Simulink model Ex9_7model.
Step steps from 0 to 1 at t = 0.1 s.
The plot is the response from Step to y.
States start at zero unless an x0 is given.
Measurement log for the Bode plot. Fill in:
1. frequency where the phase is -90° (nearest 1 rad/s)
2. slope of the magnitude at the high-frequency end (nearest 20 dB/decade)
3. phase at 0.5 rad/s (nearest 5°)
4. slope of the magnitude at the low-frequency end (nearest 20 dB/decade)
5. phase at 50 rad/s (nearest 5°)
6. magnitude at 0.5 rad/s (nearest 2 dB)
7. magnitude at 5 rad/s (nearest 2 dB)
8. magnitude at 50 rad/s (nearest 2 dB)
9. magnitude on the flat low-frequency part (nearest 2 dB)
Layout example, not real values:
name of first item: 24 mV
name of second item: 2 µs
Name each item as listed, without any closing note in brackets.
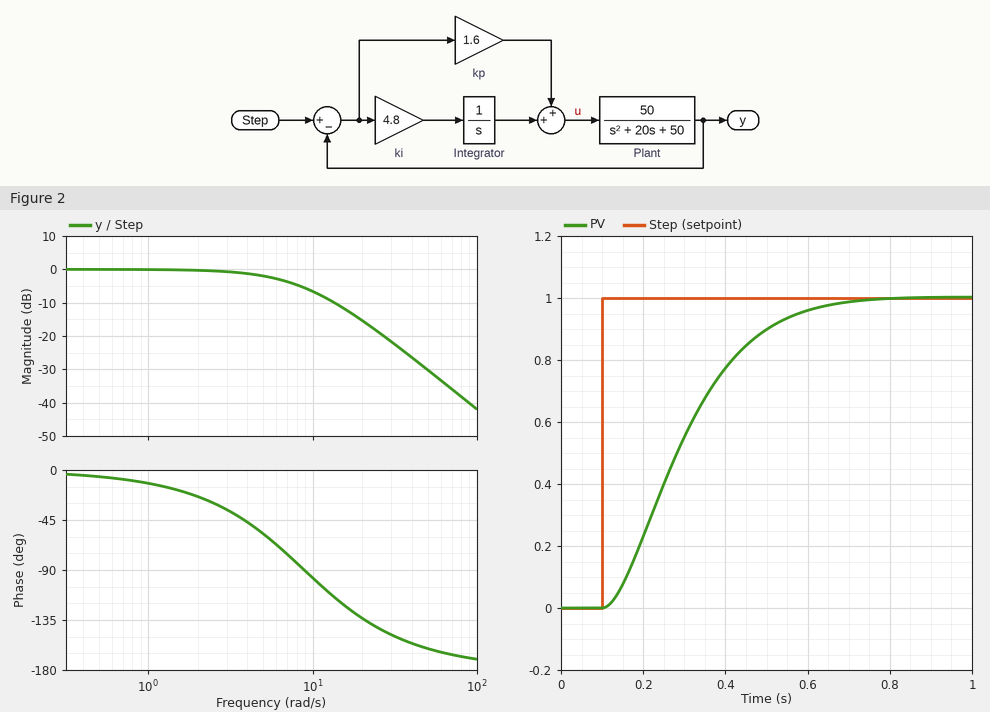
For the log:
frequency where the phase is -90°: 9 rad/s
slope of the magnitude at the high-frequency end: -40 dB/decade
phase at 0.5 rad/s: -5°
slope of the magnitude at the low-frequency end: 0 dB/decade
phase at 50 rad/s: -160°
magnitude at 0.5 rad/s: 0 dB
magnitude at 5 rad/s: -2 dB
magnitude at 50 rad/s: -30 dB
magnitude on the flat low-frequency part: 0 dB
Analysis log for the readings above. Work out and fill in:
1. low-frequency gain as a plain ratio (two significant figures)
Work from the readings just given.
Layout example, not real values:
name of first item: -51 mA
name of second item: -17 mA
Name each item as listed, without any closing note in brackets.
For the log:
low-frequency gain as a plain ratio: 1.0
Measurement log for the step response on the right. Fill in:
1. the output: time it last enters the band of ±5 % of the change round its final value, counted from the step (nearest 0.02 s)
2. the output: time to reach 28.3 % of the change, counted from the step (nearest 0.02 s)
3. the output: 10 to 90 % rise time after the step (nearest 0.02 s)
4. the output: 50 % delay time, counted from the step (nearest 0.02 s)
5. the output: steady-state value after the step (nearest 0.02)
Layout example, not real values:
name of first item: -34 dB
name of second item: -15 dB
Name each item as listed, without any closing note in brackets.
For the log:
the output: time it last enters the band of ±5 % of the change round its final value, counted from the step: 0.48 s
the output: time to reach 28.3 % of the change, counted from the step: 0.12 s
the output: 10 to 90 % rise time after the step: 0.34 s
the output: 50 % delay time, counted from the step: 0.18 s
the output: steady-state value after the step: 1.00
